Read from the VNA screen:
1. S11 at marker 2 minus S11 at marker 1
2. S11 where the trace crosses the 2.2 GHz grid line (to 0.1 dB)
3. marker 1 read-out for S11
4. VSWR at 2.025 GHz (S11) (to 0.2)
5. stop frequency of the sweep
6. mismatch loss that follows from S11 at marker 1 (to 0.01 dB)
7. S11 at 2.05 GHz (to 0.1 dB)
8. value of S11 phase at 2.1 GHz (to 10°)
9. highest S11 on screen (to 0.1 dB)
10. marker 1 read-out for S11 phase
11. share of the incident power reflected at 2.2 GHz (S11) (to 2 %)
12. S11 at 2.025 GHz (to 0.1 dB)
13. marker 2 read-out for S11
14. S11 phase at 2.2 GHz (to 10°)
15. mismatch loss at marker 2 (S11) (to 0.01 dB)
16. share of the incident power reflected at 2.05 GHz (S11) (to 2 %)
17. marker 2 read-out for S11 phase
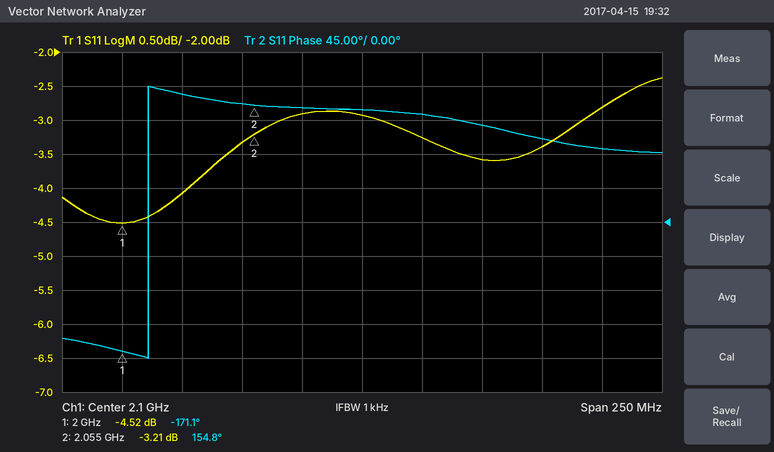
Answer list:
1.31 dB
-2.8 dB
-4.52 dB
4.4
2.225 GHz
1.89 dB
-3.3 dB
150°
-2.4 dB
-171.1°
52 %
-4.1 dB
-3.21 dB
100°
2.82 dB
46 %
154.8°
